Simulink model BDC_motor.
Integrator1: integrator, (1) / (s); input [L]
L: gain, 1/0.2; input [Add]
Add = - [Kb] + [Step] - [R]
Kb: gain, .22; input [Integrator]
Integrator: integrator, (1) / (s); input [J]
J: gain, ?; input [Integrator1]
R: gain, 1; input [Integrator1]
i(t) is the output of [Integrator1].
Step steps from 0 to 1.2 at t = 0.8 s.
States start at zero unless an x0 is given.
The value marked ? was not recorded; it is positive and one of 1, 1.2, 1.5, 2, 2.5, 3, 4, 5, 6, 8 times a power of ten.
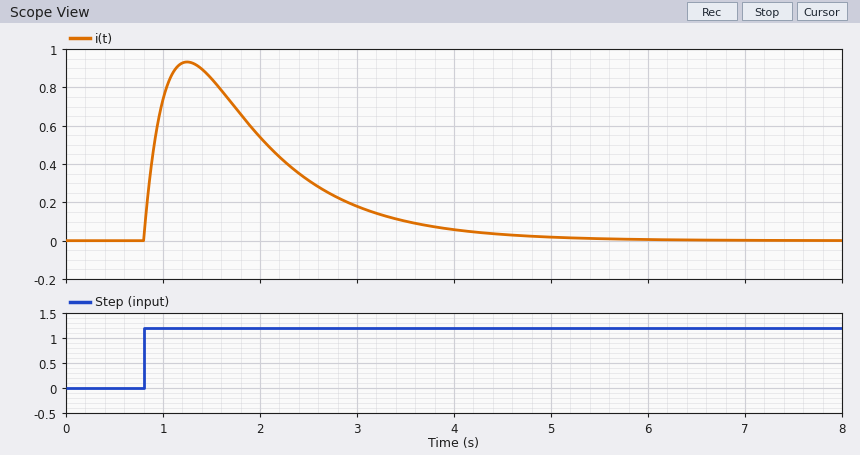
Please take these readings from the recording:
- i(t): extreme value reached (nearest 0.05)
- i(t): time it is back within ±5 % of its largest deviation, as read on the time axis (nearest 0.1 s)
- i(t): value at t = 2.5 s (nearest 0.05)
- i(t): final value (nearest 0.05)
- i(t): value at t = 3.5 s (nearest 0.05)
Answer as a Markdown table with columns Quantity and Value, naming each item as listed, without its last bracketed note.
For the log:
| Quantity | Value |
|---|---|
| i(t): extreme value reached | 0.95 |
| i(t): time it is back within ±5 % of its largest deviation, as read on the time axis | 4.2 s |
| i(t): value at t = 2.5 s | 0.30 |
| i(t): final value | 0.00 |
| i(t): value at t = 3.5 s | 0.10 |
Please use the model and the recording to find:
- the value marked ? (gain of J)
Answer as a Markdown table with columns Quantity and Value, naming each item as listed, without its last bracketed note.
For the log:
| Quantity | Value |
|---|---|
| the value marked ? | 4 |
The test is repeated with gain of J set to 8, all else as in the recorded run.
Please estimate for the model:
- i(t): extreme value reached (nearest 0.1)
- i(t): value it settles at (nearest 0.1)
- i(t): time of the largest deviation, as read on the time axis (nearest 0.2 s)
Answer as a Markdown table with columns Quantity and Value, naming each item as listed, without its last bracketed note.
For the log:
| Quantity | Value |
|---|---|
| i(t): extreme value reached | 0.8 |
| i(t): value it settles at | 0.0 |
| i(t): time of the largest deviation, as read on the time axis | 1.2 s |
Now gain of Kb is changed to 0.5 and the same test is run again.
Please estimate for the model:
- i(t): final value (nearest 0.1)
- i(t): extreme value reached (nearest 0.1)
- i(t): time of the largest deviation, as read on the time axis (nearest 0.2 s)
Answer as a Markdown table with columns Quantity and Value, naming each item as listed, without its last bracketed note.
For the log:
| Quantity | Value |
|---|---|
| i(t): final value | 0.0 |
| i(t): extreme value reached | 0.8 |
| i(t): time of the largest deviation, as read on the time axis | 1.2 s |
